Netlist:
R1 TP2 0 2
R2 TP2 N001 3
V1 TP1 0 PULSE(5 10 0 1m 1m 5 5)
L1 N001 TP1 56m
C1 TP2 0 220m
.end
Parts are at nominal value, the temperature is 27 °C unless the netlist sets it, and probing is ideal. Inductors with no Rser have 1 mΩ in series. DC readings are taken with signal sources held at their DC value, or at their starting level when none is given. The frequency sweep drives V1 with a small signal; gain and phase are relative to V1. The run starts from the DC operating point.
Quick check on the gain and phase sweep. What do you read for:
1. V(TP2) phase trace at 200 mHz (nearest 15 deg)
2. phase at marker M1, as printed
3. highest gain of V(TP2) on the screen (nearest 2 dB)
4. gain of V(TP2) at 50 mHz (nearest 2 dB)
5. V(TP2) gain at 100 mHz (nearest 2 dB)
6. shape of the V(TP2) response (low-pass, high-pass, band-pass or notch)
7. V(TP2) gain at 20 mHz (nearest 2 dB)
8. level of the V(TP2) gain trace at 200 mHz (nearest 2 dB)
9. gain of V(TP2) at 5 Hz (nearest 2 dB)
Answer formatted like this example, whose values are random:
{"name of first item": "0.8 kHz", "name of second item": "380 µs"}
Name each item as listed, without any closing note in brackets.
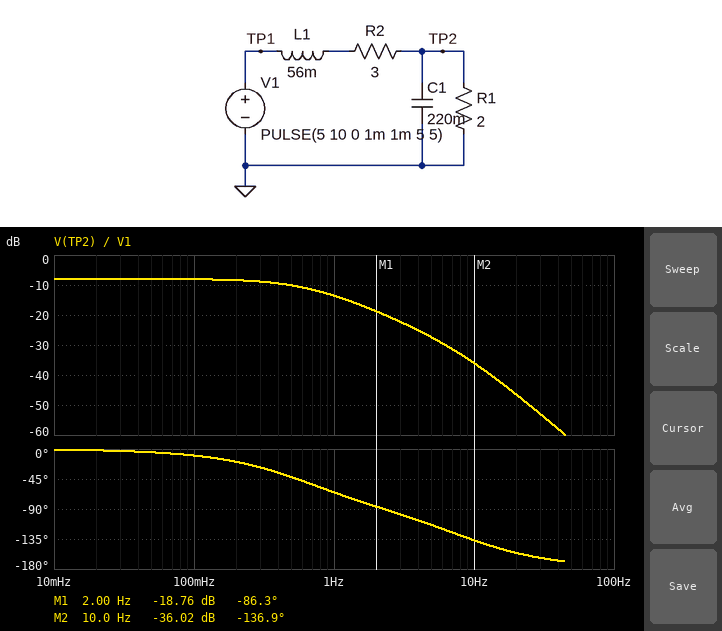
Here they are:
{"V(TP2) phase trace at 200 mHz": "-15 deg", "phase at marker M1, as printed": "-86.3 deg", "highest gain of V(TP2) on the screen": "-8 dB", "gain of V(TP2) at 50 mHz": "-8 dB", "V(TP2) gain at 100 mHz": "-8 dB", "shape of the V(TP2) response": "low-pass", "V(TP2) gain at 20 mHz": "-8 dB", "level of the V(TP2) gain trace at 200 mHz": "-8 dB", "gain of V(TP2) at 5 Hz": "-28 dB"}
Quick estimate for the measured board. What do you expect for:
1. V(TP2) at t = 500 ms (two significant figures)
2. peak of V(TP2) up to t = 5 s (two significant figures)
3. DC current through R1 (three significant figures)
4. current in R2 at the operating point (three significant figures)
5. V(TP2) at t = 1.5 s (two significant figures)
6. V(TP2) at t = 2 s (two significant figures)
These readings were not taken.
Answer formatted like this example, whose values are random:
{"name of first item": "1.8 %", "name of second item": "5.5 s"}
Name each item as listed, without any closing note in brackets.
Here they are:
{"V(TP2) at t = 500 ms": "3.7 V", "peak of V(TP2) up to t = 5 s": "4.0 V", "DC current through R1": "1.00 A", "current in R2 at the operating point": "1.00 A", "V(TP2) at t = 1.5 s": "4.0 V", "V(TP2) at t = 2 s": "4.0 V"}
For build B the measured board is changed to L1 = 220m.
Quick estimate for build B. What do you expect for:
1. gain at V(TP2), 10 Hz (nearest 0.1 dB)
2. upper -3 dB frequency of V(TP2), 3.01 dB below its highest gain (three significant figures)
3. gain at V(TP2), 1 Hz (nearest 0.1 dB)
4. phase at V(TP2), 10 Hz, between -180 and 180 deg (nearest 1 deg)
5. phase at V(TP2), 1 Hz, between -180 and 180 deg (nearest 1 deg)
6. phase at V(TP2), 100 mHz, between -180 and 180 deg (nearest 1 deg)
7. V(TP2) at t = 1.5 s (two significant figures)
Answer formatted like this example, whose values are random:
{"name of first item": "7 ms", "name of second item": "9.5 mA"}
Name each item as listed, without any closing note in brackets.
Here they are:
{"gain at V(TP2), 10 Hz": "-45.8 dB", "upper -3 dB frequency of V(TP2), 3.01 dB below its highest gain": "638 mHz", "gain at V(TP2), 1 Hz": "-13.8 dB", "phase at V(TP2), 10 Hz, between -180 and 180 deg": "-166 deg", "phase at V(TP2), 1 Hz, between -180 and 180 deg": "-83 deg", "phase at V(TP2), 100 mHz, between -180 and 180 deg": "-11 deg", "V(TP2) at t = 1.5 s": "4.0 V"}
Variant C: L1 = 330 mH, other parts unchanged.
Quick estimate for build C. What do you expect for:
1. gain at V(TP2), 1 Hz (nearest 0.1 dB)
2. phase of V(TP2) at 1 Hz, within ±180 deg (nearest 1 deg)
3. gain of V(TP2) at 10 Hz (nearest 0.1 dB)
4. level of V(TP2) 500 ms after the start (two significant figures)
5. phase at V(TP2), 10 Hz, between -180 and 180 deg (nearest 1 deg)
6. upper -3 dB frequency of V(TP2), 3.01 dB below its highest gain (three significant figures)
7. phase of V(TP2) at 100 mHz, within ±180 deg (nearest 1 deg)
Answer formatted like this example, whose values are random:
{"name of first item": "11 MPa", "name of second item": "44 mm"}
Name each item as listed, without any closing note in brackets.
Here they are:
{"gain at V(TP2), 1 Hz": "-14.3 dB", "phase of V(TP2) at 1 Hz, within ±180 deg": "-94 deg", "gain of V(TP2) at 10 Hz": "-49.2 dB", "level of V(TP2) 500 ms after the start": "3.6 V", "phase at V(TP2), 10 Hz, between -180 and 180 deg": "-170 deg", "upper -3 dB frequency of V(TP2), 3.01 dB below its highest gain": "629 mHz", "phase of V(TP2) at 100 mHz, within ±180 deg": "-12 deg"}
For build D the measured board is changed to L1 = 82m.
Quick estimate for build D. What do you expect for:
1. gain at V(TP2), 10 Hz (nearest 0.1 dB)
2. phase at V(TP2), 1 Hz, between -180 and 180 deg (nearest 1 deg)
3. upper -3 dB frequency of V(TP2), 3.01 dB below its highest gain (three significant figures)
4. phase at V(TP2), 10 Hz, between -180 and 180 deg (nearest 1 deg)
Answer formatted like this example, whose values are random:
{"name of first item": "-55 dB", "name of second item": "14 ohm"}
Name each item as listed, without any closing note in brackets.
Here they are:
{"gain at V(TP2), 10 Hz": "-38.2 dB", "phase at V(TP2), 1 Hz, between -180 and 180 deg": "-68 deg", "upper -3 dB frequency of V(TP2), 3.01 dB below its highest gain": "624 mHz", "phase at V(TP2), 10 Hz, between -180 and 180 deg": "-147 deg"}
